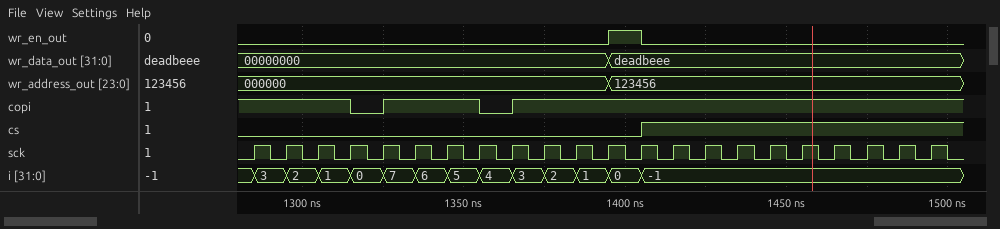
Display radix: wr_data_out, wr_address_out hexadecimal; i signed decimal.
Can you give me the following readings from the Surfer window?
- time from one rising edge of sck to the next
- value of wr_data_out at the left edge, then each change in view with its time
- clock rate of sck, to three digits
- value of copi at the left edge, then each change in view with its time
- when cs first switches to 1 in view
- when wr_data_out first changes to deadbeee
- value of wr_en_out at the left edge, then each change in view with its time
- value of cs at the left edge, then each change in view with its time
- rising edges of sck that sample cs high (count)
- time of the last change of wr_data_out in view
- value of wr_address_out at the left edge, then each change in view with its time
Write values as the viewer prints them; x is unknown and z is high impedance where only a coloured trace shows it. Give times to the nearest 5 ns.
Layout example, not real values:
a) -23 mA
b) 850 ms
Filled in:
a) 10 ns
b) 00000000, deadbeee at 1395 ns
c) 100 MHz
d) 1, 0 at 1315 ns, 1 at 1325 ns, 0 at 1355 ns, 1 at 1365 ns
e) 1405 ns
f) 1395 ns
g) 0, 1 at 1395 ns, 0 at 1405 ns
h) 0, 1 at 1405 ns
i) 9
j) 1395 ns
k) 000000, 123456 at 1395 ns
